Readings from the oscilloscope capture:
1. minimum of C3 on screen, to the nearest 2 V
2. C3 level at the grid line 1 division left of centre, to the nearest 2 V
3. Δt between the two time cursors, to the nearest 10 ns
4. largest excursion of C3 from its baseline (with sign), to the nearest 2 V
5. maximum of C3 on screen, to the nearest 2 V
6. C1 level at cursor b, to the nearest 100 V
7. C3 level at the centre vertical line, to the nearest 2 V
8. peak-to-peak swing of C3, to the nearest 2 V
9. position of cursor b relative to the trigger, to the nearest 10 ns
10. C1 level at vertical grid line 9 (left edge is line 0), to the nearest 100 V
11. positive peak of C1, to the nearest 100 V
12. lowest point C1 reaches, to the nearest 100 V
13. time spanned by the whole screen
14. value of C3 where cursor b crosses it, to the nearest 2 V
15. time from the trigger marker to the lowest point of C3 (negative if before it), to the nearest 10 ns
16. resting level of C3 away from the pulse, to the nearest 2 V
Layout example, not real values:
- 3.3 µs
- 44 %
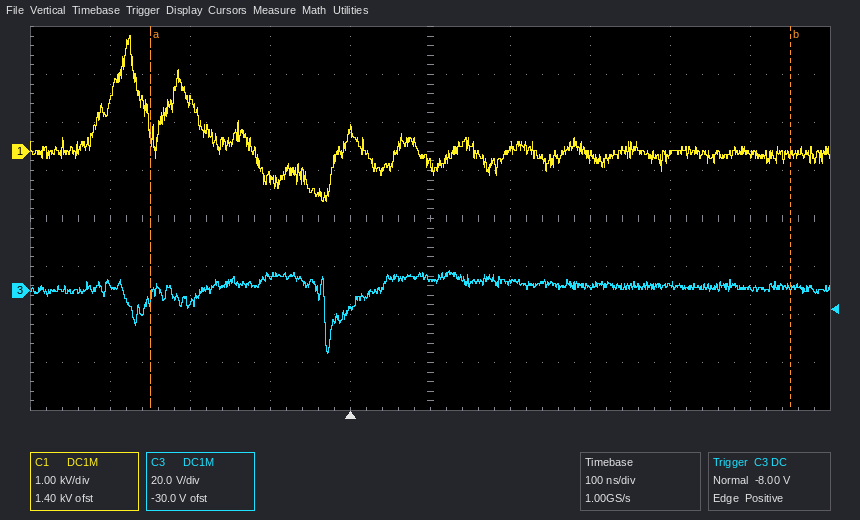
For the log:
- -26 V
- -8 V
- 800 ns
- -28 V
- 8 V
- -100 V
- 6 V
- 34 V
- +550 ns
- -100 V
- 2.4 kV
- -1.0 kV
- 1 µs
- 2 V
- -30 ns
- 2 V
